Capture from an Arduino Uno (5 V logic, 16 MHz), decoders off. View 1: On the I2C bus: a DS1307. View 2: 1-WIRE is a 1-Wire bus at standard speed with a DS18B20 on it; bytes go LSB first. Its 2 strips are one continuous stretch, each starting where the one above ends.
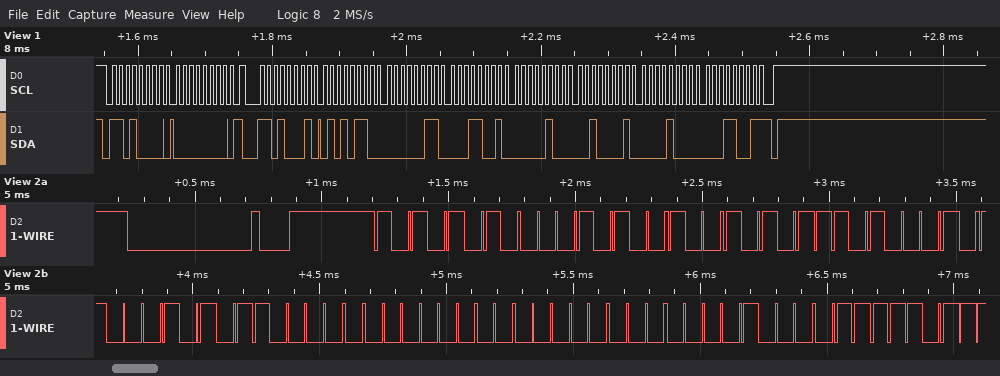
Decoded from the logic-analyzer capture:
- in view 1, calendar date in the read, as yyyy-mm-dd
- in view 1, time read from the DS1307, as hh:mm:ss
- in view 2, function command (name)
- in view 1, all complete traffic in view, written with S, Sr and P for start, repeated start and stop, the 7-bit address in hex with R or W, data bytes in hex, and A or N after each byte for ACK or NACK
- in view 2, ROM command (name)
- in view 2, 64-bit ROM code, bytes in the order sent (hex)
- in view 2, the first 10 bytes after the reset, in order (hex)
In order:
2019-08-21
19:03:56
Read Scratchpad
S 68W A 00 A Sr 68R A 56 A 03 A 19 A 04 A 21 A 08 A 19 N P
Match ROM
28 A9 8B A2 06 00 00 10
55 28 A9 8B A2 06 00 00 10 BE
